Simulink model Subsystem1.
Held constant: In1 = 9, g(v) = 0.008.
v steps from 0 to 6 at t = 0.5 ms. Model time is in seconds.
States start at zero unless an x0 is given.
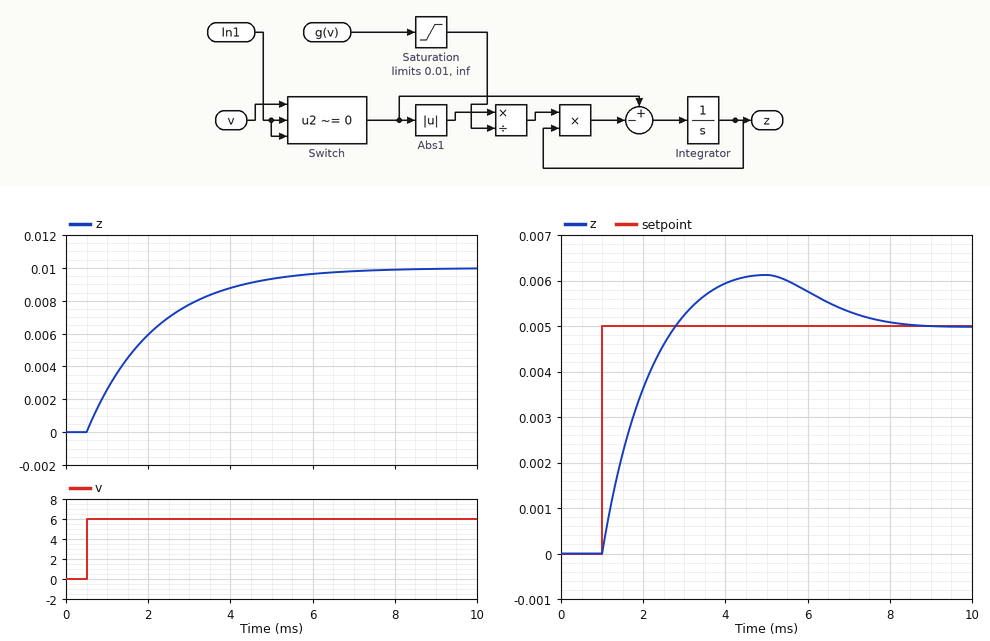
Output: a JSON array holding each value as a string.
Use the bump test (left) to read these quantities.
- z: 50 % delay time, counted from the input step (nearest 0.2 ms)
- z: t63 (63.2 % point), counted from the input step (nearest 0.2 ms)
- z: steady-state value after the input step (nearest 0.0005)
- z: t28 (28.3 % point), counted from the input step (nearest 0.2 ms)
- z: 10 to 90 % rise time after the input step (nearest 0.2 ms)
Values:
["1.2 ms", "1.6 ms", "0.0100", "0.6 ms", "3.6 ms"]
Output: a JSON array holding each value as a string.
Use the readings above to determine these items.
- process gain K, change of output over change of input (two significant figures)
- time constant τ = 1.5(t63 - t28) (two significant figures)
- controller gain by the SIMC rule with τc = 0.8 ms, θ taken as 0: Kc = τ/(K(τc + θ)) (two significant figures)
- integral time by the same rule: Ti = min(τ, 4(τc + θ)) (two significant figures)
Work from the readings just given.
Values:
["0.0017", "1.5 ms", "1100", "1.5 ms"]
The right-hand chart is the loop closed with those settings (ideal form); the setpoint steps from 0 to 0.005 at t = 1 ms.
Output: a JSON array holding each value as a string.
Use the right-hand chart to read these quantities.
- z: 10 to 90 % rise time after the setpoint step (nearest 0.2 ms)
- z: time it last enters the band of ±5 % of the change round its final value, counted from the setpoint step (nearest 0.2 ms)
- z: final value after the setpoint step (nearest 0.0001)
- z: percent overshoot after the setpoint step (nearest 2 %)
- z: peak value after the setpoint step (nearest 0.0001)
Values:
["1.4 ms", "6.2 ms", "0.0050", "22 %", "0.0061"]
